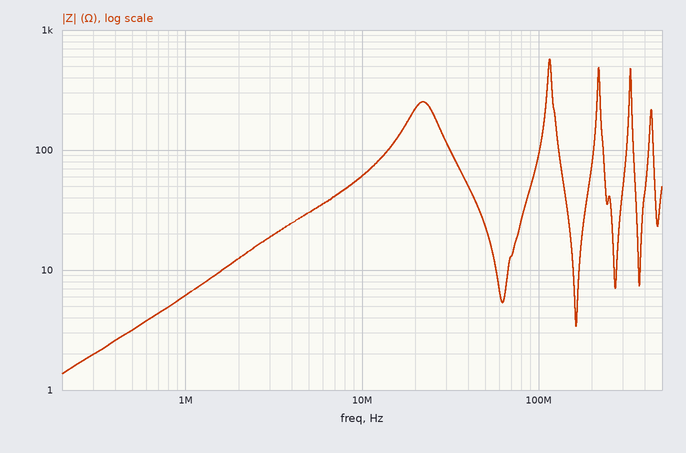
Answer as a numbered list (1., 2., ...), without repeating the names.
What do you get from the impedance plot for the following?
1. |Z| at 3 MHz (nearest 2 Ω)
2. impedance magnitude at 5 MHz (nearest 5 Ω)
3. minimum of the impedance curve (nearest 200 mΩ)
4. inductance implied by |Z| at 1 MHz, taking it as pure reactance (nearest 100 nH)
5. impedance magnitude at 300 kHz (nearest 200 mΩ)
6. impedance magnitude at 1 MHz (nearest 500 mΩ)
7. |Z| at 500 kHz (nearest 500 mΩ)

1. 18 Ω
2. 30 Ω
3. 1.4 Ω
4. 1.0 µH
5. 2.0 Ω
6. 6.0 Ω
7. 3.0 Ω
